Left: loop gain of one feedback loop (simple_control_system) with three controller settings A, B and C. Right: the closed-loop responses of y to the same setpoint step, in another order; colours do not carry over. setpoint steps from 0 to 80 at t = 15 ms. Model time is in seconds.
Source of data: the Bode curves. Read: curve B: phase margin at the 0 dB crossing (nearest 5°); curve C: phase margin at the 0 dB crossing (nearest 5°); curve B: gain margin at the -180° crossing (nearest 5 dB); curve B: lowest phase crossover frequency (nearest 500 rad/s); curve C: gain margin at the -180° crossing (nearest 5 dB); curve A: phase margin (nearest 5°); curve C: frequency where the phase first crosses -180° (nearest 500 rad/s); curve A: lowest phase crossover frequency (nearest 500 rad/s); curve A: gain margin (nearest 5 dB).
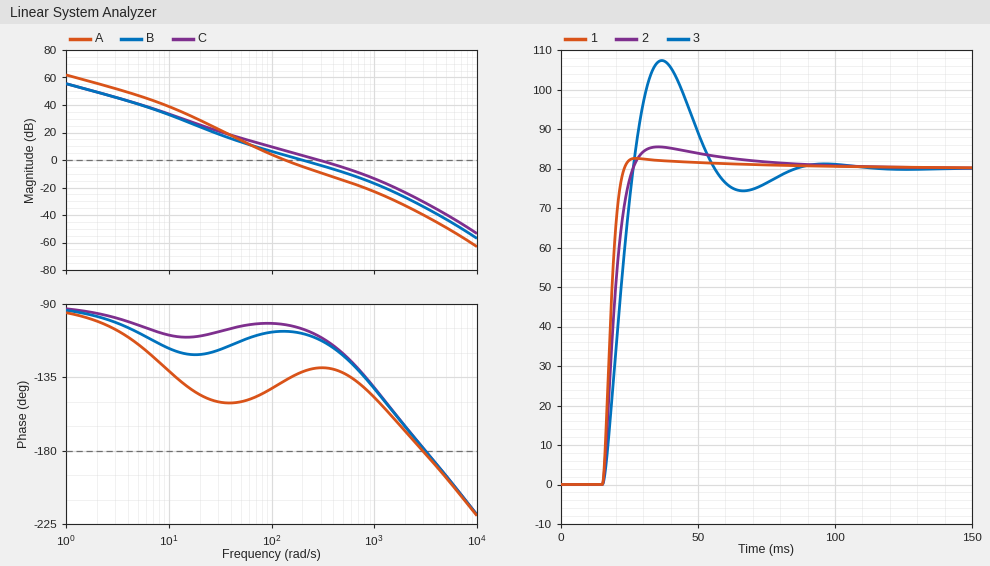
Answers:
70°
70°
35 dB
3000 rad/s
30 dB
45°
3000 rad/s
3000 rad/s
40 dB
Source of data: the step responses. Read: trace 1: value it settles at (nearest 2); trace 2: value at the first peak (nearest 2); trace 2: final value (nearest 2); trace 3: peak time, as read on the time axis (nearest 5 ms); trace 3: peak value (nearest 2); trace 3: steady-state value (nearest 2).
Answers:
80
86
80
35 ms
108
80
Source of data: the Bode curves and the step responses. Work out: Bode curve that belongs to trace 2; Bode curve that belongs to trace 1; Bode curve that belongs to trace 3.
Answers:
B
C
A
